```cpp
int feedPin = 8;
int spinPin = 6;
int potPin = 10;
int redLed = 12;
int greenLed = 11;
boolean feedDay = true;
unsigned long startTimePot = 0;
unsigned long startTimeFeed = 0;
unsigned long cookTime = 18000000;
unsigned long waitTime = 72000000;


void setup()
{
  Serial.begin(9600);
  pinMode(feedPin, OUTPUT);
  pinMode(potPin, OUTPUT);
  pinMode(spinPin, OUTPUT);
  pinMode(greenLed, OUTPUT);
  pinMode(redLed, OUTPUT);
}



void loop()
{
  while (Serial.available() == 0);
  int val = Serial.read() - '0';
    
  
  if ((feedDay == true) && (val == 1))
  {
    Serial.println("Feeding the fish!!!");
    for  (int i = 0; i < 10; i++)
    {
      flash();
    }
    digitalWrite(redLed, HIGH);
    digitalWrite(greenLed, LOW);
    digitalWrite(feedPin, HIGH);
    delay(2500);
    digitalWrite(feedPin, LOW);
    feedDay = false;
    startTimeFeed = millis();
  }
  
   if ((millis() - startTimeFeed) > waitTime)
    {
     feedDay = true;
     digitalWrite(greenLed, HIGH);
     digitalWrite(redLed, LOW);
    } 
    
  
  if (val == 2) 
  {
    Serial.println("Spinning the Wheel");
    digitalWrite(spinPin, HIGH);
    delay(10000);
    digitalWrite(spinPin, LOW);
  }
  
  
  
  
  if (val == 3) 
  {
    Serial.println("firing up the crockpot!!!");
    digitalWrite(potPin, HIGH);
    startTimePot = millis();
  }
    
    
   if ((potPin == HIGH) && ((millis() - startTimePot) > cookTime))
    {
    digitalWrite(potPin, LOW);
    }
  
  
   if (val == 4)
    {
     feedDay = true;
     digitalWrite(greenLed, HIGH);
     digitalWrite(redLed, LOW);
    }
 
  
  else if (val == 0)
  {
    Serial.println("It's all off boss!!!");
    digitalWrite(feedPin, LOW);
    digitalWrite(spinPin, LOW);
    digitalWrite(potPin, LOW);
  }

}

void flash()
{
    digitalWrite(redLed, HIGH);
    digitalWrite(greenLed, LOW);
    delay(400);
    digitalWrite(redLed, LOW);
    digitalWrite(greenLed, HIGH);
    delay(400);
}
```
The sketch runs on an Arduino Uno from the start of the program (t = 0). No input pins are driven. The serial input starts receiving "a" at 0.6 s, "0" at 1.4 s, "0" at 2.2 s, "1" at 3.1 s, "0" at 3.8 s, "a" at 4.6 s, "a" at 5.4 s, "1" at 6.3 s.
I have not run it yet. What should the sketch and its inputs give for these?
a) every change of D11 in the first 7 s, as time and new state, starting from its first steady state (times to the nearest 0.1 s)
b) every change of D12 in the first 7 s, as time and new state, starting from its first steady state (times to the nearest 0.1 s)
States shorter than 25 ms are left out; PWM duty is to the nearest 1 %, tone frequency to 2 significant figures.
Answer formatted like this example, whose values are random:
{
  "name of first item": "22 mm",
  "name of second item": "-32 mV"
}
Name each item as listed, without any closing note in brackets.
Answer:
{
  "every change of D11 in the first 7 s, as time and new state, starting from its first steady state": "0 s low; 3.5 s high; 3.9 s low; 4.3 s high; 4.7 s low; 5.1 s high; 5.5 s low; 5.9 s high; 6.3 s low; 6.7 s high",
  "every change of D12 in the first 7 s, as time and new state, starting from its first steady state": "0 s low; 3.1 s high; 3.5 s low; 3.9 s high; 4.3 s low; 4.7 s high; 5.1 s low; 5.5 s high; 5.9 s low; 6.3 s high; 6.7 s low"
}
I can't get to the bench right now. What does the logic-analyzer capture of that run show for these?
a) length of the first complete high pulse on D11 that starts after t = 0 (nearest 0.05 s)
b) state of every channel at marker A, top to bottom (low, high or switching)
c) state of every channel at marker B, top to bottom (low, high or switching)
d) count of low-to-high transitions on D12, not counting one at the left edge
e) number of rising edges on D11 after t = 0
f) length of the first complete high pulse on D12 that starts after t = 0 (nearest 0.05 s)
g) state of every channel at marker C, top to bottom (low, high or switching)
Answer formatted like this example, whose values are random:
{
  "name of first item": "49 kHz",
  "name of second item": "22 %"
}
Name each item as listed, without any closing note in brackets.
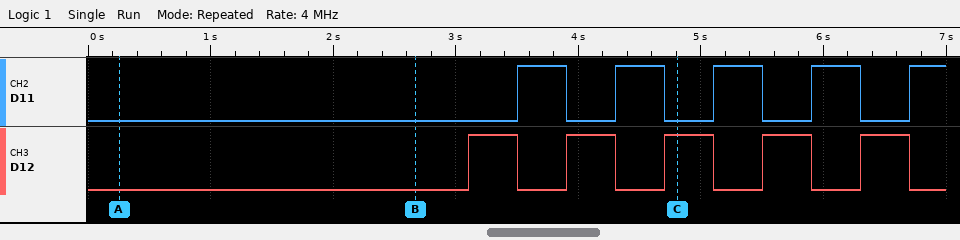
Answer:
{
  "length of the first complete high pulse on D11 that starts after t = 0": "0.40 s",
  "state of every channel at marker A, top to bottom": "D11 low, D12 low",
  "state of every channel at marker B, top to bottom": "D11 low, D12 low",
  "count of low-to-high transitions on D12, not counting one at the left edge": "5",
  "number of rising edges on D11 after t = 0": "5",
  "length of the first complete high pulse on D12 that starts after t = 0": "0.40 s",
  "state of every channel at marker C, top to bottom": "D11 low, D12 high"
}
